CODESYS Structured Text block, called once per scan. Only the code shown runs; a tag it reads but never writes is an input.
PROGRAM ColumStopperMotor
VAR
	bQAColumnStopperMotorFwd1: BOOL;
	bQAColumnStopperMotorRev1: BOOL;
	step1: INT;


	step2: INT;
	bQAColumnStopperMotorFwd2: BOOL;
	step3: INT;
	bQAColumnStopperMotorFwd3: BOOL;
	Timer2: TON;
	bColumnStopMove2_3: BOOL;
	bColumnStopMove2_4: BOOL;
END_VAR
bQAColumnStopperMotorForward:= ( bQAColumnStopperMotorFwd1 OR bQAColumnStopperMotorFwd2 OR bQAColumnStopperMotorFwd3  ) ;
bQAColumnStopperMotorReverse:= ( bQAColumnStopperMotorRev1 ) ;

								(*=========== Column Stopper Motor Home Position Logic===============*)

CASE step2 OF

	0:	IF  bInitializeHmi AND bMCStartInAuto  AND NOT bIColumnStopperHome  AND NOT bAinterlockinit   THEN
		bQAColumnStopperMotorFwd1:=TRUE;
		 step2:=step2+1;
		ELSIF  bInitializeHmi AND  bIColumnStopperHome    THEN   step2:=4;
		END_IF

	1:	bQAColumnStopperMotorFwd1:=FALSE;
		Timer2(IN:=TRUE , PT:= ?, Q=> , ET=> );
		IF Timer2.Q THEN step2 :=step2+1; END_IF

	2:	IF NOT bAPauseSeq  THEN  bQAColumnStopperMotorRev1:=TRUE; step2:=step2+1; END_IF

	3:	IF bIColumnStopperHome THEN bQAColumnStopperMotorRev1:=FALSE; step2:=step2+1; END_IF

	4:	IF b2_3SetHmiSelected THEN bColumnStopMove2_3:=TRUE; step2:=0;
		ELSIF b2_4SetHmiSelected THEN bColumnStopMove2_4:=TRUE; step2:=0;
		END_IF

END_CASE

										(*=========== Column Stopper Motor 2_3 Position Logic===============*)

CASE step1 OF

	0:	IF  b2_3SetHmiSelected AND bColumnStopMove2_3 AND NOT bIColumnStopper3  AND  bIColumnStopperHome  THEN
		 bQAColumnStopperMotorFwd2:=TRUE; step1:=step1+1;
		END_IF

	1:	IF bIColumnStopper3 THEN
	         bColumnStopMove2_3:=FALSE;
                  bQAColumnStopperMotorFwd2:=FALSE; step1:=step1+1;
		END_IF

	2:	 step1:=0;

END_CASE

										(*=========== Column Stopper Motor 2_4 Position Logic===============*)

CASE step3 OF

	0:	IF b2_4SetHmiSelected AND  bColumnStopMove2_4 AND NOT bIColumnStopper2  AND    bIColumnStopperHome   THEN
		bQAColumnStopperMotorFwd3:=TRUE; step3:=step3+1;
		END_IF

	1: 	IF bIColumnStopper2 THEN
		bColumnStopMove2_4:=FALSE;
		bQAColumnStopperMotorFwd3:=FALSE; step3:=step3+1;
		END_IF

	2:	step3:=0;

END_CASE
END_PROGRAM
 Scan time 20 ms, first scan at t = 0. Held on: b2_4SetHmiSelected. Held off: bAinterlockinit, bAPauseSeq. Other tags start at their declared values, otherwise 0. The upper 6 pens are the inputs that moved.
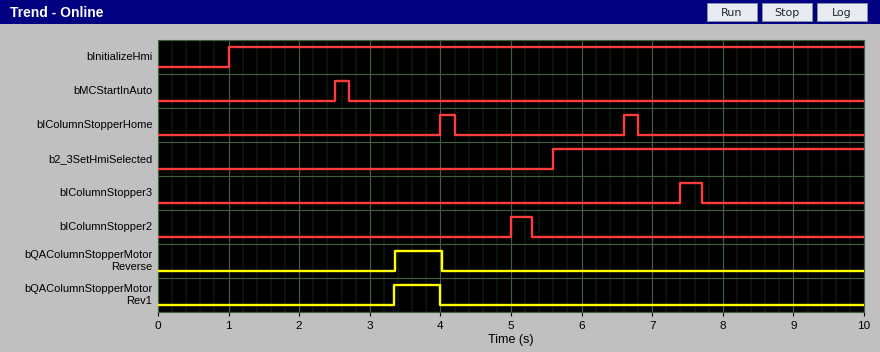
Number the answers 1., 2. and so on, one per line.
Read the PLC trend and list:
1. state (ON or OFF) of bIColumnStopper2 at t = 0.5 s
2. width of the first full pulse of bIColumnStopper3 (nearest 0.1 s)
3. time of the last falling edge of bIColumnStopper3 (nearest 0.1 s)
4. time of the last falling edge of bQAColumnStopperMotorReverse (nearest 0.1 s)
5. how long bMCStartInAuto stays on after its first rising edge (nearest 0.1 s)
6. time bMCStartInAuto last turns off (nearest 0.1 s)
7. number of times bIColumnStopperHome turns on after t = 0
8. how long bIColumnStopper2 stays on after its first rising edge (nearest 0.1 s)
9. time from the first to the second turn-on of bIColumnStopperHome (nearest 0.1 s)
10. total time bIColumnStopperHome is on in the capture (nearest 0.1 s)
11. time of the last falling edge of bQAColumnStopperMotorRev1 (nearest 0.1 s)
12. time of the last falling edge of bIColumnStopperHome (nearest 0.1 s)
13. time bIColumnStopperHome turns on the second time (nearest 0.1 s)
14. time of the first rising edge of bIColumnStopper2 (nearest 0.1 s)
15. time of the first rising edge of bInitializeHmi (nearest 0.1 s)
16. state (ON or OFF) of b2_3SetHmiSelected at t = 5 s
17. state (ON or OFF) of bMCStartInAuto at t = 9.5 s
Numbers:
1. OFF
2. 0.3 s
3. 7.7 s
4. 4.0 s
5. 0.2 s
6. 2.7 s
7. 2
8. 0.3 s
9. 2.6 s
10. 0.4 s
11. 4.0 s
12. 6.8 s
13. 6.6 s
14. 5.0 s
15. 1.0 s
16. OFF
17. OFF
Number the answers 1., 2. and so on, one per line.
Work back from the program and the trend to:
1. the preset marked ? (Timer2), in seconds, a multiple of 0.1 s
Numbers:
1. 0.8 s
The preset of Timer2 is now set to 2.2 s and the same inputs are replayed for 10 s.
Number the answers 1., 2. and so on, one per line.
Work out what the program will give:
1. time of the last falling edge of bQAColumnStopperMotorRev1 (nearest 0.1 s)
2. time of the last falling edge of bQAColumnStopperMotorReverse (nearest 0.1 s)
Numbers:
1. 6.6 s
2. 6.6 s
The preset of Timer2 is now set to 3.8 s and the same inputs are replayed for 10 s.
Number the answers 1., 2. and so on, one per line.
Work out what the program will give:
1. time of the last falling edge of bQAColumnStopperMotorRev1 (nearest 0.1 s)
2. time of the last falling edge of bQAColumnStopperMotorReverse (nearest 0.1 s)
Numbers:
1. 6.6 s
2. 6.6 s
